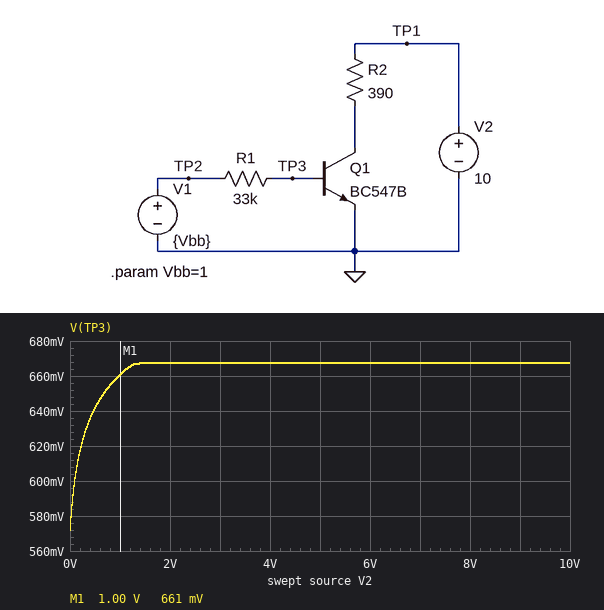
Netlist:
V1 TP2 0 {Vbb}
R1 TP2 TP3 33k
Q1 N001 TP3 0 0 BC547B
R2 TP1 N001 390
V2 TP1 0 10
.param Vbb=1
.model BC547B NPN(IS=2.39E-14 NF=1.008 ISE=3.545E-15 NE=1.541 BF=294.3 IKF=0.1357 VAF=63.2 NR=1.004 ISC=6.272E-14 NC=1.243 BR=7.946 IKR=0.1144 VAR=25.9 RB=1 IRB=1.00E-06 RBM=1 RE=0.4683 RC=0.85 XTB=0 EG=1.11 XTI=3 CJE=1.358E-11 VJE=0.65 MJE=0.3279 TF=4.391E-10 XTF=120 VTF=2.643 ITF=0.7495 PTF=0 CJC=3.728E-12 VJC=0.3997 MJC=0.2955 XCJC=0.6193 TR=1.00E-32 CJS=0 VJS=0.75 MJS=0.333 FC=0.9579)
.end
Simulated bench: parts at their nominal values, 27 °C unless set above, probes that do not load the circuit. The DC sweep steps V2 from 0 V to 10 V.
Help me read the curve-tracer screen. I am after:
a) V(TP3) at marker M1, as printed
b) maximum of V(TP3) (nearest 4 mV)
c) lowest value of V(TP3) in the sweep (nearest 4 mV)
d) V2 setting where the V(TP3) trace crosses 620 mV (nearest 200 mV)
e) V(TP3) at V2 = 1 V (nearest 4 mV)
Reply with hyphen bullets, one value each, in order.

- 661 mV
- 668 mV
- 572 mV
- 200 mV
- 660 mV
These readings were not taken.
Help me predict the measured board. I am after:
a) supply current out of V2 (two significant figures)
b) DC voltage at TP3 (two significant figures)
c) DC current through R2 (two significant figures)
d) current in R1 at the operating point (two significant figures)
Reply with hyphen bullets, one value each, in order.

- 3.2 mA
- 670 mV
- 3.2 mA
- 10 µA
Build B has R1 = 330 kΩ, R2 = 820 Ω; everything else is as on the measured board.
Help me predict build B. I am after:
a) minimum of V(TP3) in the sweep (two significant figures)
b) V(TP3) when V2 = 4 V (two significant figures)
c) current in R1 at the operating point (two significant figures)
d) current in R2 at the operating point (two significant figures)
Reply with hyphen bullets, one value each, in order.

- 510 mV
- 610 mV
- 1.2 µA
- 380 µA
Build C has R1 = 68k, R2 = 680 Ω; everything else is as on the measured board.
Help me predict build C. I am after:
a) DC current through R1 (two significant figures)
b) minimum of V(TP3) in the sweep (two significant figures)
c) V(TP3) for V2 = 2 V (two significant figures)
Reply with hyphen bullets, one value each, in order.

- 5.2 µA
- 550 mV
- 650 mV
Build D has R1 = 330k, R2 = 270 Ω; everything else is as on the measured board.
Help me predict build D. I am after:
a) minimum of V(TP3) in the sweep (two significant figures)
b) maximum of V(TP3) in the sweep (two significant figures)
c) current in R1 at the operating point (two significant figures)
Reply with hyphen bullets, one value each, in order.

- 510 mV
- 610 mV
- 1.2 µA
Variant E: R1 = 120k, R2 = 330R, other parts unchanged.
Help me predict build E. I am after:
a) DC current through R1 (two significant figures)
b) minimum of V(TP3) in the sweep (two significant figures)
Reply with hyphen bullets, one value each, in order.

- 3.0 µA
- 540 mV
